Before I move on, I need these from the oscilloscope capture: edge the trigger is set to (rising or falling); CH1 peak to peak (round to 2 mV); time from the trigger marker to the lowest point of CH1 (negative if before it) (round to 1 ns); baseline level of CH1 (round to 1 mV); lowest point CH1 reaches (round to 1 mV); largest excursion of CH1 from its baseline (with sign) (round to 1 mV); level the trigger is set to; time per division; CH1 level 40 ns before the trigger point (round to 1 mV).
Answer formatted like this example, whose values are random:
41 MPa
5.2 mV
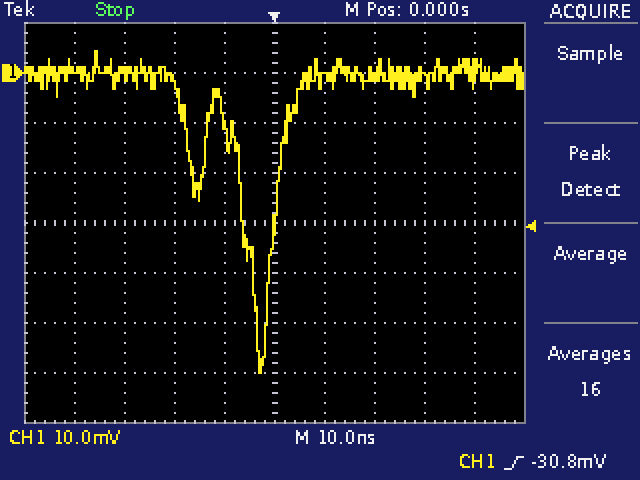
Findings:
rising
64 mV
-3 ns
-1 mV
-60 mV
-59 mV
-30.8 mV
10 ns
1 mV
